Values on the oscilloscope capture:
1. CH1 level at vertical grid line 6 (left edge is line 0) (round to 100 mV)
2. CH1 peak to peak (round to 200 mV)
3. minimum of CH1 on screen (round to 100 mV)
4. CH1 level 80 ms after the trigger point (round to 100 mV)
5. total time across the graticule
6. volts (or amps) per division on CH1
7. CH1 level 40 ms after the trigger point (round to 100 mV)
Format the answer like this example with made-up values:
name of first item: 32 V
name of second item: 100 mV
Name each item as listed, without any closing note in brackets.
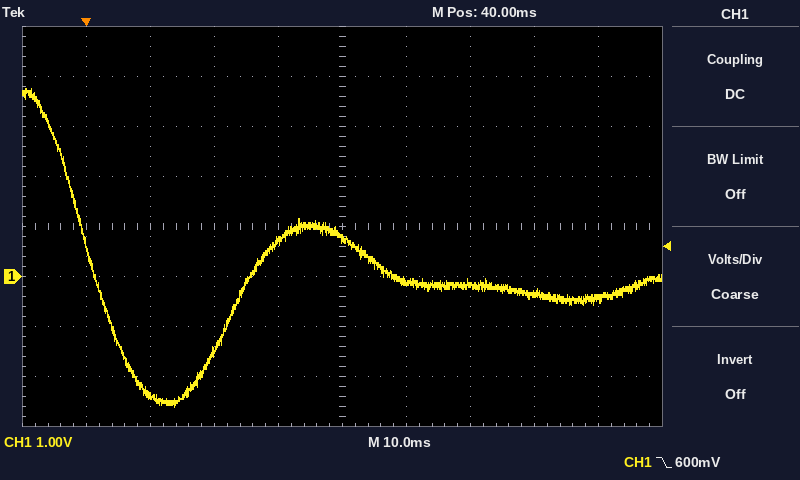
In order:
CH1 level at vertical grid line 6 (left edge is line 0): -100 mV
CH1 peak to peak: 6.4 V
minimum of CH1 on screen: -2.6 V
CH1 level 80 ms after the trigger point: -400 mV
total time across the graticule: 100 ms
volts (or amps) per division on CH1: 1 V
CH1 level 40 ms after the trigger point: 800 mV
